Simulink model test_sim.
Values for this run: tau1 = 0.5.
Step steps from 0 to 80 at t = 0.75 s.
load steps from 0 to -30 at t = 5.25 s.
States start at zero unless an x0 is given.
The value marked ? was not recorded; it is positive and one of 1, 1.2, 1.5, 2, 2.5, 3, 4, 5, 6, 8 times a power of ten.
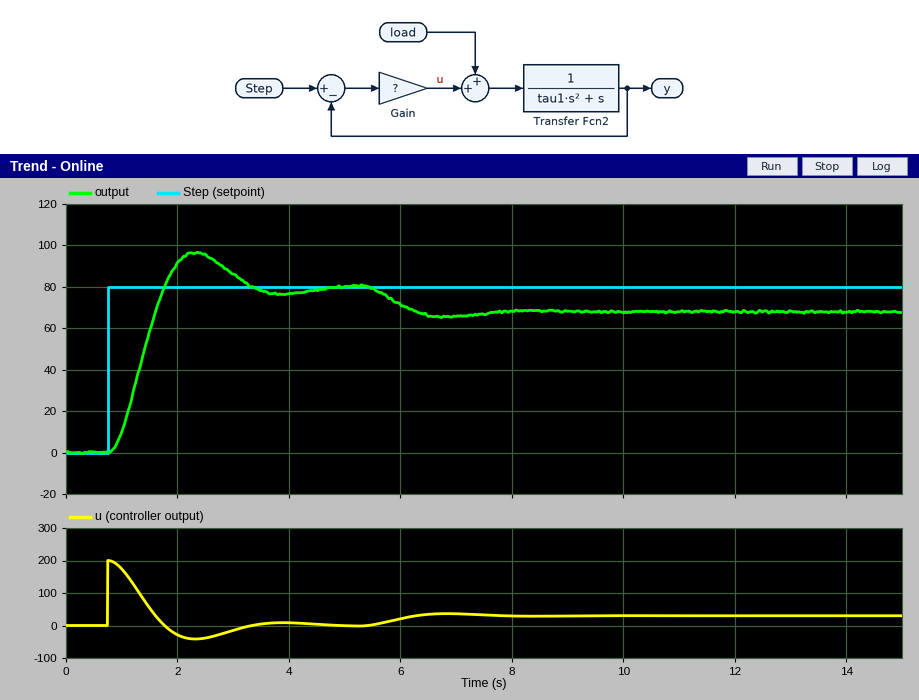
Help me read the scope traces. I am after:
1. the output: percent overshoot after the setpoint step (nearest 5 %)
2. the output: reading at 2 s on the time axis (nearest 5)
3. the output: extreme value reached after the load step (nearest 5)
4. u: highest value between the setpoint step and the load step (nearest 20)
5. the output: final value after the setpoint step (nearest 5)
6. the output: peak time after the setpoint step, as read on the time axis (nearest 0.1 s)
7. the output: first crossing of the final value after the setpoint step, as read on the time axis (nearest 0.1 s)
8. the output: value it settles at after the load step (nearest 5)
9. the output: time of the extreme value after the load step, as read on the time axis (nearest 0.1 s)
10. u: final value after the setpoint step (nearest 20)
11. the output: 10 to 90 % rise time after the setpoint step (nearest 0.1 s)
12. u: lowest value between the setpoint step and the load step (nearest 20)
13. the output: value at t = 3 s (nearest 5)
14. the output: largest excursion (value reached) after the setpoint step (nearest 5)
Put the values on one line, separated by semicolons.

20 %; 90; 65; 200; 80; 2.3 s; 1.8 s; 70; 6.8 s; 0; 0.7 s; -40; 85; 95
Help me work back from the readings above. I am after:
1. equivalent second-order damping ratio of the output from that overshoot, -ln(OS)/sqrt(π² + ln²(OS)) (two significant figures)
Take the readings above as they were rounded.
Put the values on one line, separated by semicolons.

0.46
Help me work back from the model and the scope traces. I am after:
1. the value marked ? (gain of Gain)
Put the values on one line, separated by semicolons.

2.5
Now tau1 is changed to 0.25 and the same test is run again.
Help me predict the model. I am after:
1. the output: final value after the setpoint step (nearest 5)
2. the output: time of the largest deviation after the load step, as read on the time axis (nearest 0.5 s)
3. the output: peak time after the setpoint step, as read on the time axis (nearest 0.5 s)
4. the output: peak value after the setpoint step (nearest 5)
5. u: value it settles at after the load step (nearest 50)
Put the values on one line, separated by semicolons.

80; 6.5 s; 2.0 s; 85; 50
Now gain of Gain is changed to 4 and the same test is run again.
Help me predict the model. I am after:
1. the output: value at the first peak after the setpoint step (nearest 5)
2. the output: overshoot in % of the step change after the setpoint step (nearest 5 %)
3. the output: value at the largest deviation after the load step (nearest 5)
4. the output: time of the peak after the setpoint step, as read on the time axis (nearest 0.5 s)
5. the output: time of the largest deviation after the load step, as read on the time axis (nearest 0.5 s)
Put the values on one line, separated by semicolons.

105; 30 %; 70; 2.0 s; 6.5 s
